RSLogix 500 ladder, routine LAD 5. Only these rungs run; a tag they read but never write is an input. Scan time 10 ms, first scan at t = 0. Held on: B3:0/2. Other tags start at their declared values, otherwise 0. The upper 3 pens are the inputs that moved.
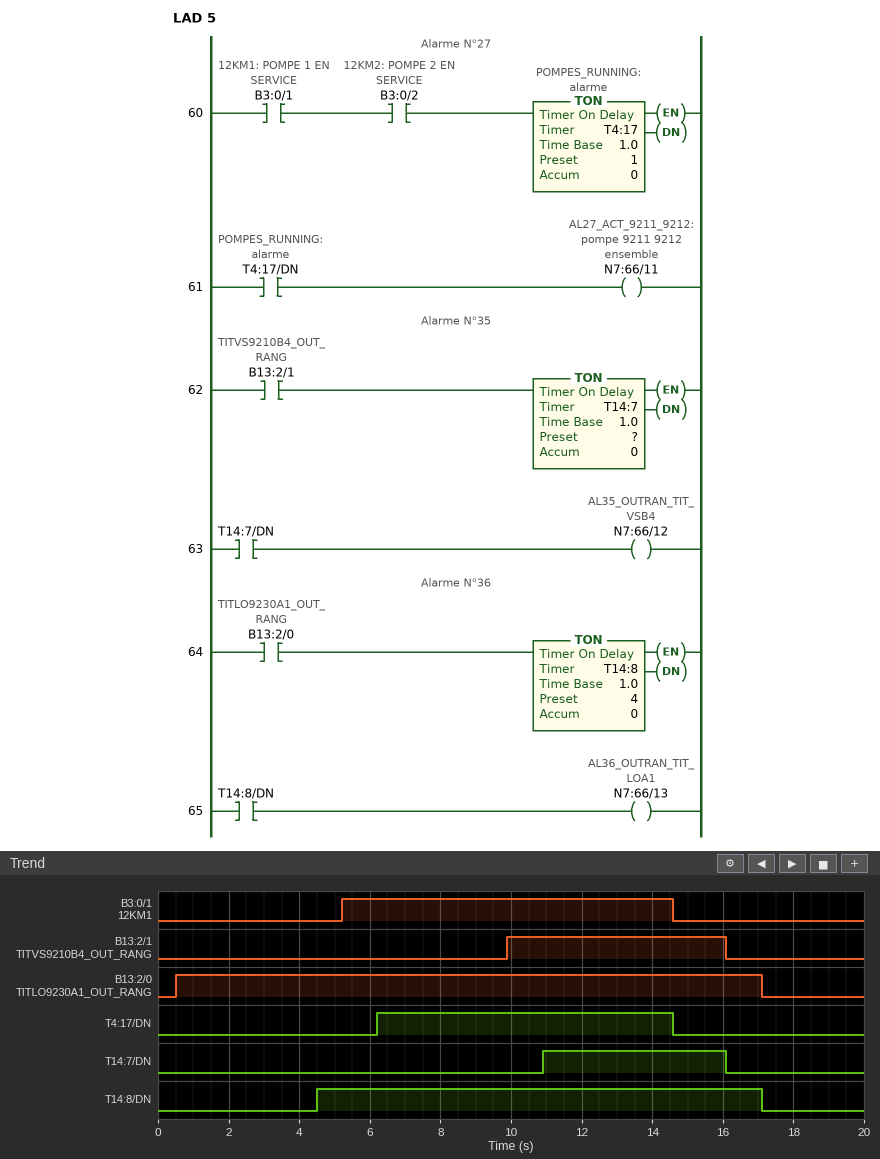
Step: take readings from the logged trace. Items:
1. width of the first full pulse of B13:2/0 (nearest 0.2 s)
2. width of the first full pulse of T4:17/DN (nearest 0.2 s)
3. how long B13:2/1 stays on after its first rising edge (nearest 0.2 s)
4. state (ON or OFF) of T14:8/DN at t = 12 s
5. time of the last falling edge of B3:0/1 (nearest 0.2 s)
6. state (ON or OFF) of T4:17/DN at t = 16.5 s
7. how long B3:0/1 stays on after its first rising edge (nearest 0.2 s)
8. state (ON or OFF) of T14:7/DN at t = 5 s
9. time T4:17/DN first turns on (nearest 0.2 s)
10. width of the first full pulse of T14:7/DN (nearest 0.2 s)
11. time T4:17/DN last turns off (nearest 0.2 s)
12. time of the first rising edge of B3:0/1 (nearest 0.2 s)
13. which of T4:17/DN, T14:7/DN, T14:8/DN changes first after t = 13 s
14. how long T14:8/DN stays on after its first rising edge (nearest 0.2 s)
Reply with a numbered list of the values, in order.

1. 16.6 s
2. 8.4 s
3. 6.2 s
4. ON
5. 14.6 s
6. OFF
7. 9.4 s
8. OFF
9. 6.2 s
10. 5.2 s
11. 14.6 s
12. 5.2 s
13. T4:17/DN
14. 12.6 s
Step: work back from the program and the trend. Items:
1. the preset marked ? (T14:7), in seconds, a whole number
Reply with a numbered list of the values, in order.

1. 1 s
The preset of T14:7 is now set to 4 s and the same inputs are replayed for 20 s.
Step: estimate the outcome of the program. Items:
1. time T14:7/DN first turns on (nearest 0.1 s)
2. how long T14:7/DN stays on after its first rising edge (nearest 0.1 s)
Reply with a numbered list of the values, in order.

1. 13.9 s
2. 2.2 s
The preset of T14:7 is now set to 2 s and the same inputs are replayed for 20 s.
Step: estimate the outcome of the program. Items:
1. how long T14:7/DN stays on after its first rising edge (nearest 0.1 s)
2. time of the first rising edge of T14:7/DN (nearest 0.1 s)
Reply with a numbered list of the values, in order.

1. 4.2 s
2. 11.9 s
